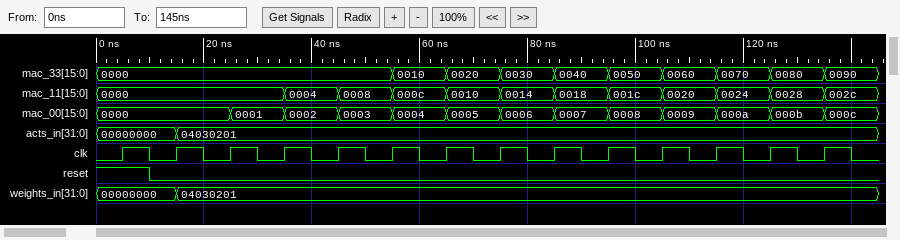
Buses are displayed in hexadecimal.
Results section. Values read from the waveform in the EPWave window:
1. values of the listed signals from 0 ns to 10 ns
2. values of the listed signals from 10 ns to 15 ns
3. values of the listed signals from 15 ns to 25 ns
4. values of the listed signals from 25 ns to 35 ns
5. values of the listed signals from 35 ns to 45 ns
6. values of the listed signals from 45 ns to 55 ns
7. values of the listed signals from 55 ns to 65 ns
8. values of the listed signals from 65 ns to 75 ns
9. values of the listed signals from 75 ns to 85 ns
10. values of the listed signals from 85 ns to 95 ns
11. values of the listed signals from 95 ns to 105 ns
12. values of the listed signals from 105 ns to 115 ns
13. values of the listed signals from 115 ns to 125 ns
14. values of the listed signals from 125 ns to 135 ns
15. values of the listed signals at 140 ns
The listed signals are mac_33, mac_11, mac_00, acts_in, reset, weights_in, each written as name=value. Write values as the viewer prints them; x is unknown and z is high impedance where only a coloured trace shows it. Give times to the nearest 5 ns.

mac_33=0000, mac_11=0000, mac_00=0000, acts_in=00000000, reset=1, weights_in=00000000
mac_33=0000, mac_11=0000, mac_00=0000, acts_in=00000000, reset=0, weights_in=00000000
mac_33=0000, mac_11=0000, mac_00=0000, acts_in=04030201, reset=0, weights_in=04030201
mac_33=0000, mac_11=0000, mac_00=0001, acts_in=04030201, reset=0, weights_in=04030201
mac_33=0000, mac_11=0004, mac_00=0002, acts_in=04030201, reset=0, weights_in=04030201
mac_33=0000, mac_11=0008, mac_00=0003, acts_in=04030201, reset=0, weights_in=04030201
mac_33=0010, mac_11=000c, mac_00=0004, acts_in=04030201, reset=0, weights_in=04030201
mac_33=0020, mac_11=0010, mac_00=0005, acts_in=04030201, reset=0, weights_in=04030201
mac_33=0030, mac_11=0014, mac_00=0006, acts_in=04030201, reset=0, weights_in=04030201
mac_33=0040, mac_11=0018, mac_00=0007, acts_in=04030201, reset=0, weights_in=04030201
mac_33=0050, mac_11=001c, mac_00=0008, acts_in=04030201, reset=0, weights_in=04030201
mac_33=0060, mac_11=0020, mac_00=0009, acts_in=04030201, reset=0, weights_in=04030201
mac_33=0070, mac_11=0024, mac_00=000a, acts_in=04030201, reset=0, weights_in=04030201
mac_33=0080, mac_11=0028, mac_00=000b, acts_in=04030201, reset=0, weights_in=04030201
mac_33=0090, mac_11=002c, mac_00=000c, acts_in=04030201, reset=0, weights_in=04030201
